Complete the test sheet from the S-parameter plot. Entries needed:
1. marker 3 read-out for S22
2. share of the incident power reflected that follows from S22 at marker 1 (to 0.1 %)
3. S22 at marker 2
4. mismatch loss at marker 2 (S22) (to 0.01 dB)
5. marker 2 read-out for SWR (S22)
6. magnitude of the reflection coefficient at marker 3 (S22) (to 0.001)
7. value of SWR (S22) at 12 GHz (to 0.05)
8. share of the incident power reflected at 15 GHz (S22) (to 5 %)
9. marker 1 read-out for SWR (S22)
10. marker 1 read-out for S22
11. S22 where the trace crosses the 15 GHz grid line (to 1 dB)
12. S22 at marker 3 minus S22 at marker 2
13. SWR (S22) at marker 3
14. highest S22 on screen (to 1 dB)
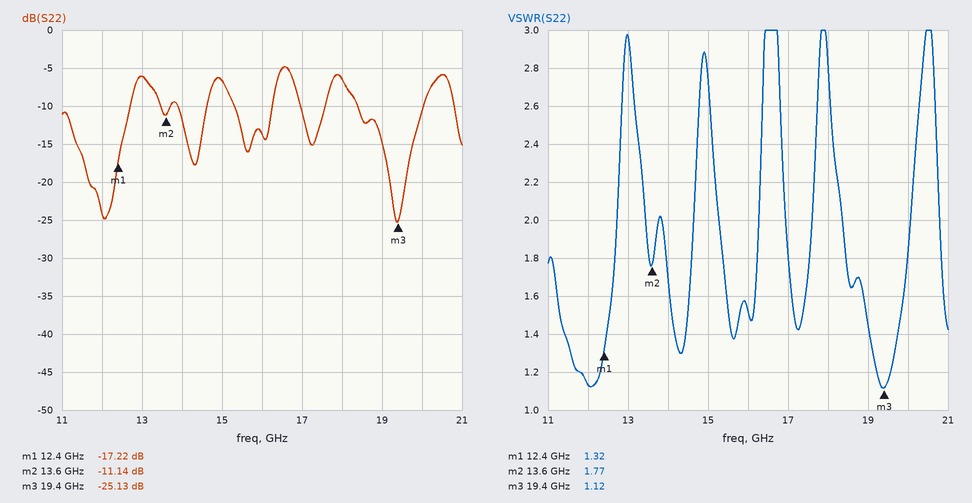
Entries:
-25.13 dB
1.9 %
-11.14 dB
0.35 dB
1.77
0.055
1.15
20 %
1.32
-17.22 dB
-7 dB
-13.99 dB
1.12
-5 dB
